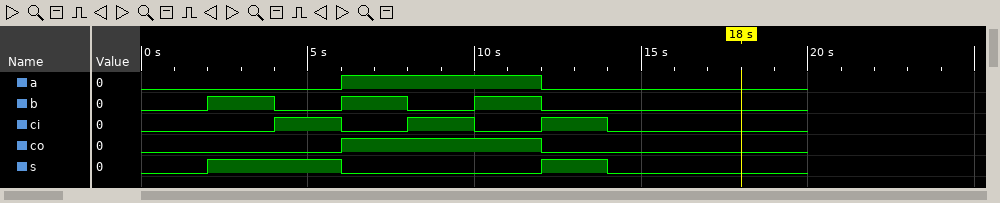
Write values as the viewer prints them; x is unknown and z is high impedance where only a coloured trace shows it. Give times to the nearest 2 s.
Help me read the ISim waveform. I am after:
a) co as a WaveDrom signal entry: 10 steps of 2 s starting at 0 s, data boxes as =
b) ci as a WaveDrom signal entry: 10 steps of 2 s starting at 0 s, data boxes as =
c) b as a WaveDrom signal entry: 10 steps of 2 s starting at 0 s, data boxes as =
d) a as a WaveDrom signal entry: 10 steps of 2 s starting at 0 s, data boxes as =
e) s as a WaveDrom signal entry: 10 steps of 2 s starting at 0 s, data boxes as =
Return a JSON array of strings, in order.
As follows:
["{name: 'co', wave: '0..1..0...'}", "{name: 'ci', wave: '0.101010..'}", "{name: 'b', wave: '0101010...'}", "{name: 'a', wave: '0..1..0...'}", "{name: 's', wave: '01.0..10..'}"]
